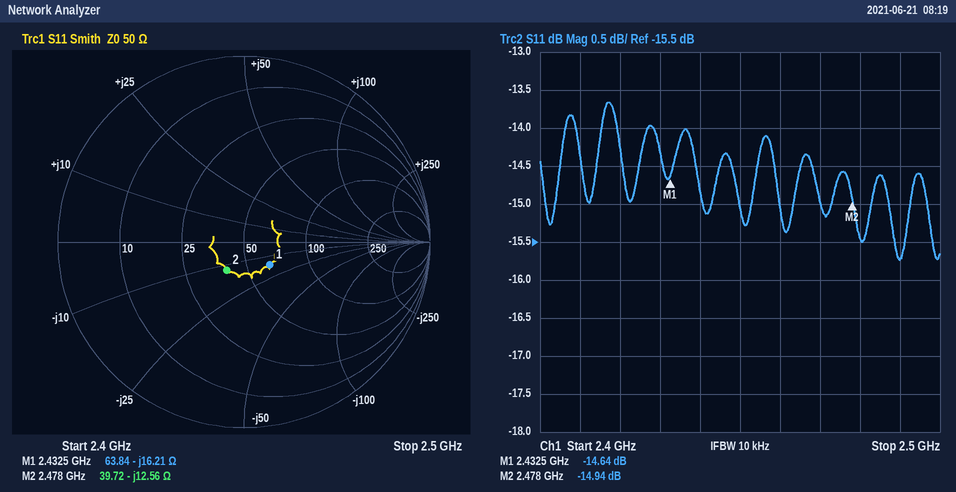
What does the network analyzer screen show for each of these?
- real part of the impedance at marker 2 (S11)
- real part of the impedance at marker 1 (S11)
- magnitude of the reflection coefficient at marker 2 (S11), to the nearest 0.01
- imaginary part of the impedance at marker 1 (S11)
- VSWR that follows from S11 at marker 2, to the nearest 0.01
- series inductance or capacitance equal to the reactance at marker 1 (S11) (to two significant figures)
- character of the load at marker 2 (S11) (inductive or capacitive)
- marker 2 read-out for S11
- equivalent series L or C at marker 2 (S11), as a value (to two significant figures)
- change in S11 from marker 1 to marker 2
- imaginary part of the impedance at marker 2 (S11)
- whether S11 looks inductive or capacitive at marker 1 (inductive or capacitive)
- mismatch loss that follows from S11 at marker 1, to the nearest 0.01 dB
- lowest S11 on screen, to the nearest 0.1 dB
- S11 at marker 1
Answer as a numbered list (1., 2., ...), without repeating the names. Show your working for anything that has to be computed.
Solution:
1. 39.72 Ω
2. 63.84 Ω
3. 0.18
4. -16.21 Ω
5. (1 + 0.1791)/(1 − 0.1791) ≈ 1.44
6. C = 1/(2π × 2.4325 GHz × 16.21 Ω) ≈ 4.0 pF
7. capacitive
8. -14.94 dB
9. C = 1/(2π × 2.478 GHz × 12.56 Ω) ≈ 5.1 pF
10. -14.94 − (-14.64) = -0.30 dB
11. -12.56 Ω
12. capacitive
13. −10 log10(1 − 10^(-14.64/10)) ≈ 0.15 dB
14. -15.7 dB
15. -14.64 dB
